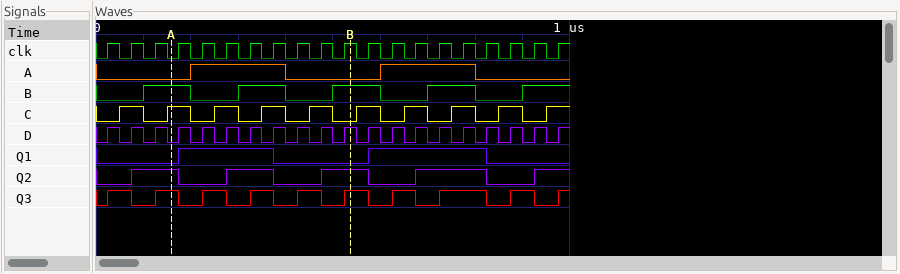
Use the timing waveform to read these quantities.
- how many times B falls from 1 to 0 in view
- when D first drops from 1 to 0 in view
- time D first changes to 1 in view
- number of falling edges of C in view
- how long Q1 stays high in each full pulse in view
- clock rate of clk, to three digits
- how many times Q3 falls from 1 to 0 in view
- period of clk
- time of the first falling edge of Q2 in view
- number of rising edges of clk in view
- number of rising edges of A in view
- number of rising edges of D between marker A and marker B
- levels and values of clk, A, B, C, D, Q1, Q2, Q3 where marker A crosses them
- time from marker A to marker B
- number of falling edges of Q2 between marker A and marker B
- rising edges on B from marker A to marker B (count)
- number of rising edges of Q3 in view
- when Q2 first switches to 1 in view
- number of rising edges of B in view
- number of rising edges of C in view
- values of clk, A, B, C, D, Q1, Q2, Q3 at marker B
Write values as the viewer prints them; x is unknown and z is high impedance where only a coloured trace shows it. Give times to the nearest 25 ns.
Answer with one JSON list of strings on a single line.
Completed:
["4", "50 ns", "25 ns", "9", "200 ns, 250 ns", "20.0 MHz", "9", "50 ns", "175 ns", "20", "2", "8", "clk=0, A=0, B=1, C=1, D=0, Q1=0, Q2=1, Q3=1", "375 ns", "2", "2", "10", "75 ns", "5", "10", "clk=1, A=0, B=1, C=0, D=1, Q1=0, Q2=1, Q3=1"]
